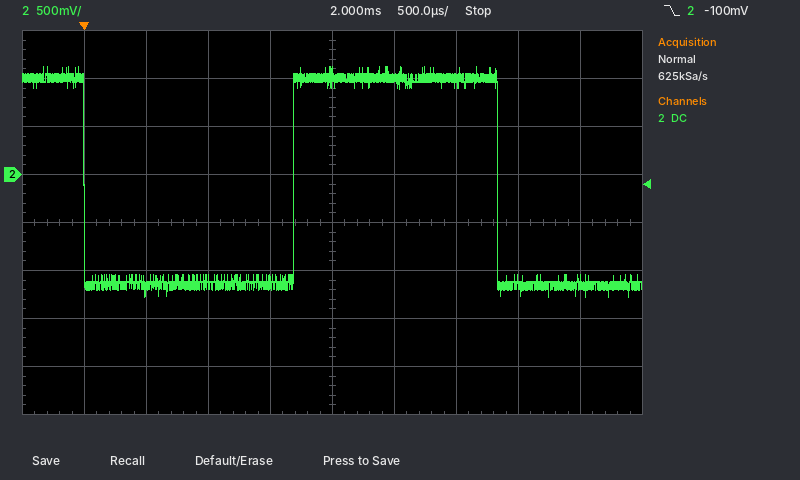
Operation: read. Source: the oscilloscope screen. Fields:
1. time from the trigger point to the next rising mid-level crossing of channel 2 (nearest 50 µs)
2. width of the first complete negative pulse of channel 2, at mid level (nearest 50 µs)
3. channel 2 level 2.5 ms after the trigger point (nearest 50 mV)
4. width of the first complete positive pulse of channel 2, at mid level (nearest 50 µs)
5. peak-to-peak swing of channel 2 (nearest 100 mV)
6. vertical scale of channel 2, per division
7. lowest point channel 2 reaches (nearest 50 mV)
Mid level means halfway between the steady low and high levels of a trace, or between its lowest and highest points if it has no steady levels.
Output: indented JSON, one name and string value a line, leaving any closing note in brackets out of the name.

{
  "time from the trigger point to the next rising mid-level crossing of channel 2": "1.70 ms",
  "width of the first complete negative pulse of channel 2, at mid level": "1.70 ms",
  "channel 2 level 2.5 ms after the trigger point": "1.00 V",
  "width of the first complete positive pulse of channel 2, at mid level": "1.65 ms",
  "peak-to-peak swing of channel 2": "2.40 V",
  "vertical scale of channel 2, per division": "500 mV",
  "lowest point channel 2 reaches": "-1.25 V"
}
